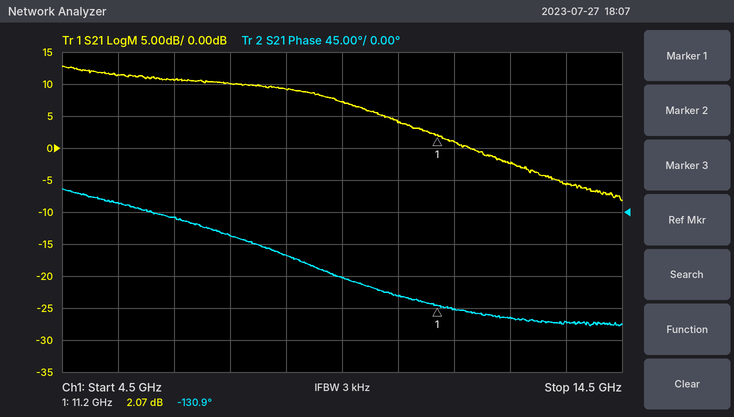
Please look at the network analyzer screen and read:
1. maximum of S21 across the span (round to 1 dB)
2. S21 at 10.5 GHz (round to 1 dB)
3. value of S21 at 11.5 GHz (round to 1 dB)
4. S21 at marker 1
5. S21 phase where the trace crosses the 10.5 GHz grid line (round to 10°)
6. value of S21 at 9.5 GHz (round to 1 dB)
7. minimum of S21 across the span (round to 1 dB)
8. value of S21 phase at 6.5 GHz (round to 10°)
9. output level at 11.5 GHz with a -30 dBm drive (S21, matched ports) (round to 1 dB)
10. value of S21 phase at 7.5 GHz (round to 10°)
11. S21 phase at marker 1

13 dB
4 dB
1 dB
2.07 dB
-120°
7 dB
-8 dB
-10°
-29 dBm
-30°
-130.9°
